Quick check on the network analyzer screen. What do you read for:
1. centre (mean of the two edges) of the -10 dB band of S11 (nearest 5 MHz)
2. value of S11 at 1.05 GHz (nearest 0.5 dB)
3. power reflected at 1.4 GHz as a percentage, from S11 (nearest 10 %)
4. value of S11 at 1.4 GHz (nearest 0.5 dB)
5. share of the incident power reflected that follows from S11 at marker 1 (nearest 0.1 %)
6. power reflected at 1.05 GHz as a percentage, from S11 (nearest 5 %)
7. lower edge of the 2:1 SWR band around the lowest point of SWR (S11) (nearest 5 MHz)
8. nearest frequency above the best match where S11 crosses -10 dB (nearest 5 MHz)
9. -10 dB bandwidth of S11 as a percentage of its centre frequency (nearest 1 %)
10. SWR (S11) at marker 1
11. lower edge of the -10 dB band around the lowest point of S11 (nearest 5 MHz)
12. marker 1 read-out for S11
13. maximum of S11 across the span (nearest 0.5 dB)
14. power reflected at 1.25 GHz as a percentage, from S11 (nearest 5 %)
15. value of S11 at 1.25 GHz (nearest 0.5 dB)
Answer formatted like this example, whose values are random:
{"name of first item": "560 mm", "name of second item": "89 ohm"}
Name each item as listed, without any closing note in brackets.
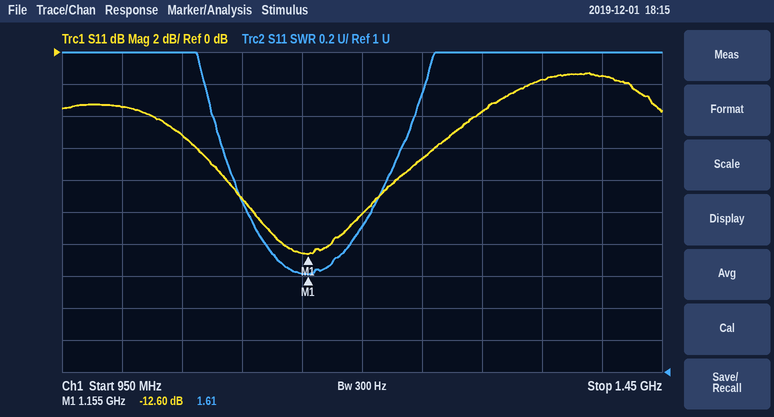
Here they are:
{"centre (mean of the two edges) of the -10 dB band of S11": "1.155 GHz", "value of S11 at 1.05 GHz": "-5.0 dB", "power reflected at 1.4 GHz as a percentage, from S11": "70 %", "value of S11 at 1.4 GHz": "-1.5 dB", "share of the incident power reflected that follows from S11 at marker 1": "5.5 %", "power reflected at 1.05 GHz as a percentage, from S11": "30 %", "lower edge of the 2:1 SWR band around the lowest point of SWR (S11)": "1.105 GHz", "nearest frequency above the best match where S11 crosses -10 dB": "1.200 GHz", "-10 dB bandwidth of S11 as a percentage of its centre frequency": "8 %", "SWR (S11) at marker 1": "1.61", "lower edge of the -10 dB band around the lowest point of S11": "1.110 GHz", "marker 1 read-out for S11": "-12.60 dB", "maximum of S11 across the span": "-1.5 dB", "power reflected at 1.25 GHz as a percentage, from S11": "20 %", "value of S11 at 1.25 GHz": "-6.5 dB"}
